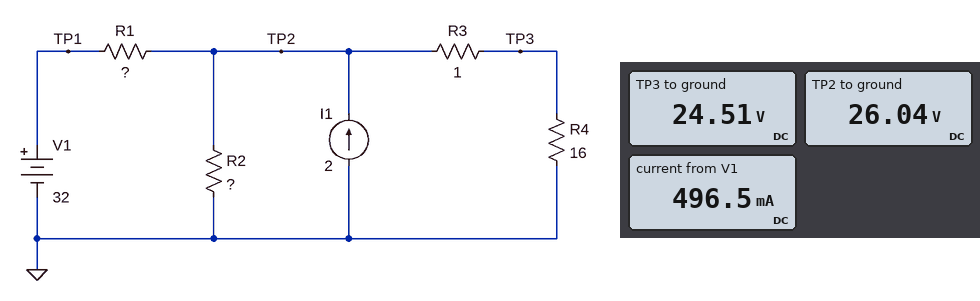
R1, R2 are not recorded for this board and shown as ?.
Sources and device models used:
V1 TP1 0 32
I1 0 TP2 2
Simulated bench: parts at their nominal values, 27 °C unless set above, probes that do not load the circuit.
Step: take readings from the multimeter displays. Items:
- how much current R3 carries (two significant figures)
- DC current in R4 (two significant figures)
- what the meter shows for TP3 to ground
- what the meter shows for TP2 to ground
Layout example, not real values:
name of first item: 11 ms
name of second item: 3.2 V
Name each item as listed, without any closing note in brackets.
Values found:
how much current R3 carries: 1.5 A
DC current in R4: 1.5 A
what the meter shows for TP3 to ground: 24.51 V
what the meter shows for TP2 to ground: 26.04 V
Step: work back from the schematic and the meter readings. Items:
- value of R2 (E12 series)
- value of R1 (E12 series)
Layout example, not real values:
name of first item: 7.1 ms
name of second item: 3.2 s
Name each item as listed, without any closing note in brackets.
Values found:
value of R2: 27 Ω
value of R1: 12 Ω
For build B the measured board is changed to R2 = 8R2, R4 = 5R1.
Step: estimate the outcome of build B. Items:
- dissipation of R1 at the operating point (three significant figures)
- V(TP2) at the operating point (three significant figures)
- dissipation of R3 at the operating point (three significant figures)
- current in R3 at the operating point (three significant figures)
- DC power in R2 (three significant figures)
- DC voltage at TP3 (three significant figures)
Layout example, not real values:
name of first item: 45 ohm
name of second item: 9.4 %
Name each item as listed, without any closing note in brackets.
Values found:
dissipation of R1 at the operating point: 31.2 W
V(TP2) at the operating point: 12.6 V
dissipation of R3 at the operating point: 4.29 W
current in R3 at the operating point: 2.07 A
DC power in R2: 19.5 W
DC voltage at TP3: 10.6 V
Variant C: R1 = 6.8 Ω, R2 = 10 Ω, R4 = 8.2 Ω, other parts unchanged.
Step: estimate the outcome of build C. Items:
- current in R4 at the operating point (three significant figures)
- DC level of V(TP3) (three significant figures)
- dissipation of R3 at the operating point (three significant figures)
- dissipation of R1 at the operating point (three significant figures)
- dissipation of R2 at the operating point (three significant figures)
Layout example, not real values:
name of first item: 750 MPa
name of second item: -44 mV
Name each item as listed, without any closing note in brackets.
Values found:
current in R4 at the operating point: 2.05 A
DC level of V(TP3): 16.8 V
dissipation of R3 at the operating point: 4.20 W
dissipation of R1 at the operating point: 25.4 W
dissipation of R2 at the operating point: 35.5 W
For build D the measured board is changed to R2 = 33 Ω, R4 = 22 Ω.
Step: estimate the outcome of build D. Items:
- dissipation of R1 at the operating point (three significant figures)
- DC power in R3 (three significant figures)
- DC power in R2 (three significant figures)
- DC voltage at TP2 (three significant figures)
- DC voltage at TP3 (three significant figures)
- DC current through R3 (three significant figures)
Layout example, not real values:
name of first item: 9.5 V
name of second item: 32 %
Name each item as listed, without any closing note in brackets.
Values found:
dissipation of R1 at the operating point: 440 mW
DC power in R3: 1.67 W
DC power in R2: 26.7 W
DC voltage at TP2: 29.7 V
DC voltage at TP3: 28.4 V
DC current through R3: 1.29 A
